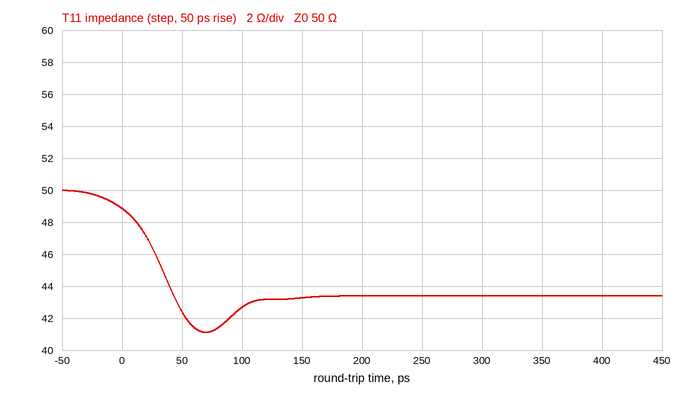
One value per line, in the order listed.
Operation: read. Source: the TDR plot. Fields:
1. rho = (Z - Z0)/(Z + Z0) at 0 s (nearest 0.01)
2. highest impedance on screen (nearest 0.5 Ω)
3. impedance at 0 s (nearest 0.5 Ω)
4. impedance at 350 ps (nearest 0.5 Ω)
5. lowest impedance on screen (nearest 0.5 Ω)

-0.01
50.0 Ω
49.0 Ω
43.5 Ω
41.0 Ω
